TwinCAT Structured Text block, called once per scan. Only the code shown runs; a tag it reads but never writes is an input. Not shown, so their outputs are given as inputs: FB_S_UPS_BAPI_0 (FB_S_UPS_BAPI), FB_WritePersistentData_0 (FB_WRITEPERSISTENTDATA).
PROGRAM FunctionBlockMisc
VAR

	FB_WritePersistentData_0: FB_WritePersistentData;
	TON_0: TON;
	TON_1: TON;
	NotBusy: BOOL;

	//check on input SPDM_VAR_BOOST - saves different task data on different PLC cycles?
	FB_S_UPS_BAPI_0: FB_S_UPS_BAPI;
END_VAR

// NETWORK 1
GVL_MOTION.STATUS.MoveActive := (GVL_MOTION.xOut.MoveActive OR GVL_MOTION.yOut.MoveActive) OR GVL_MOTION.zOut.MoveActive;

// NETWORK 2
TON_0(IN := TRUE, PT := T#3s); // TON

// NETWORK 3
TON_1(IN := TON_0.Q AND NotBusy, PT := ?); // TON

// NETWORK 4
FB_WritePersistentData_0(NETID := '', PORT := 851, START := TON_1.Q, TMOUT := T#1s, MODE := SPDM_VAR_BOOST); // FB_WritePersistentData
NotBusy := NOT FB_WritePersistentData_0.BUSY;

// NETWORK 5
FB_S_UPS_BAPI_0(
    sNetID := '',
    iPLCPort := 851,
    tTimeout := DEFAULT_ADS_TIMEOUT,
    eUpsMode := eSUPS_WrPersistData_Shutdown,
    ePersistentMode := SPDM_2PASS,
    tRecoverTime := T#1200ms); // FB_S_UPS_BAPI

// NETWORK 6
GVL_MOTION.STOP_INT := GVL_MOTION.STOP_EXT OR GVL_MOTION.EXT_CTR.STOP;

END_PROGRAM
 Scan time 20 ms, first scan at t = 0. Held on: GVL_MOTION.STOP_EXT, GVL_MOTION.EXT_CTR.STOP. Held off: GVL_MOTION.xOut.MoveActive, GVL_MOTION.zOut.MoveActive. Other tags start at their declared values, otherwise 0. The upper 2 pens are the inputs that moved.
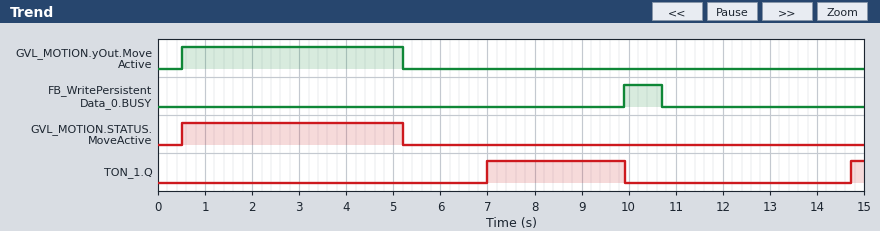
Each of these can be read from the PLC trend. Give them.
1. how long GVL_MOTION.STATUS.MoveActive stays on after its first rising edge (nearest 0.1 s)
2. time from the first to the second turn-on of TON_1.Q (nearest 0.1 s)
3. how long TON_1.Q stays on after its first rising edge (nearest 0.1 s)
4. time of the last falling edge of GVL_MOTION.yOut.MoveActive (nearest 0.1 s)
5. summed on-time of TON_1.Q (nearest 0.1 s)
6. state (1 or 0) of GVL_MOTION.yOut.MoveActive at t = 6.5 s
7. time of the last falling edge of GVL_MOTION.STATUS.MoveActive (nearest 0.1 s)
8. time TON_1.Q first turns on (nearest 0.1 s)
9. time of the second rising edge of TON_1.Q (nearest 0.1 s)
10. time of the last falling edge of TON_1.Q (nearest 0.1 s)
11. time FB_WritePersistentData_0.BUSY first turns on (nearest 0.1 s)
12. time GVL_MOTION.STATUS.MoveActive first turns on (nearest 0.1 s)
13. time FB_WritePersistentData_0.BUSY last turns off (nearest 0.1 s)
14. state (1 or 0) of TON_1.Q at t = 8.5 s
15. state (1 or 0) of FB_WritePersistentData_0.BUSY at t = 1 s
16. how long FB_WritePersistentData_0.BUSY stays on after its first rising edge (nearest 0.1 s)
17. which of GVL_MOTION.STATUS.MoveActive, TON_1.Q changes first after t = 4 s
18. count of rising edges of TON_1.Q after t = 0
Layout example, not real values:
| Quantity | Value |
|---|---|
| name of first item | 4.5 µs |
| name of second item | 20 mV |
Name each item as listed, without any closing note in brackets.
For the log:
| Quantity | Value |
|---|---|
| how long GVL_MOTION.STATUS.MoveActive stays on after its first rising edge | 4.7 s |
| time from the first to the second turn-on of TON_1.Q | 7.7 s |
| how long TON_1.Q stays on after its first rising edge | 2.9 s |
| time of the last falling edge of GVL_MOTION.yOut.MoveActive | 5.2 s |
| summed on-time of TON_1.Q | 3.2 s |
| state (1 or 0) of GVL_MOTION.yOut.MoveActive at t = 6.5 s | 0 |
| time of the last falling edge of GVL_MOTION.STATUS.MoveActive | 5.2 s |
| time TON_1.Q first turns on | 7.0 s |
| time of the second rising edge of TON_1.Q | 14.7 s |
| time of the last falling edge of TON_1.Q | 9.9 s |
| time FB_WritePersistentData_0.BUSY first turns on | 9.9 s |
| time GVL_MOTION.STATUS.MoveActive first turns on | 0.5 s |
| time FB_WritePersistentData_0.BUSY last turns off | 10.7 s |
| state (1 or 0) of TON_1.Q at t = 8.5 s | 1 |
| state (1 or 0) of FB_WritePersistentData_0.BUSY at t = 1 s | 0 |
| how long FB_WritePersistentData_0.BUSY stays on after its first rising edge | 0.8 s |
| which of GVL_MOTION.STATUS.MoveActive, TON_1.Q changes first after t = 4 s | GVL_MOTION.STATUS.MoveActive |
| count of rising edges of TON_1.Q after t = 0 | 2 |
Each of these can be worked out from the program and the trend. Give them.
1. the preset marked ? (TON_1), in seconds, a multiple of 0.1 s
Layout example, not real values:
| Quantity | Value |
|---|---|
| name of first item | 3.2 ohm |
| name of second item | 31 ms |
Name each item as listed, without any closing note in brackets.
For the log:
| Quantity | Value |
|---|---|
| the preset marked ? (TON_1), in seconds, a multiple of 0.1 s | 4.0 s |
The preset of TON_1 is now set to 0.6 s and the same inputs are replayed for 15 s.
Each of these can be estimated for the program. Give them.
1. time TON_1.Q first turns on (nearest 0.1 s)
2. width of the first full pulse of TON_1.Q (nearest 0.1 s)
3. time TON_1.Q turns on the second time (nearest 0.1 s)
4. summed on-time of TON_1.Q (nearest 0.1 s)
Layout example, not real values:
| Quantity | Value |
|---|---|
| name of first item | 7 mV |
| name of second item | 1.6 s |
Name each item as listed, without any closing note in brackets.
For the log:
| Quantity | Value |
|---|---|
| time TON_1.Q first turns on | 3.6 s |
| width of the first full pulse of TON_1.Q | 6.3 s |
| time TON_1.Q turns on the second time | 11.3 s |
| summed on-time of TON_1.Q | 10.0 s |
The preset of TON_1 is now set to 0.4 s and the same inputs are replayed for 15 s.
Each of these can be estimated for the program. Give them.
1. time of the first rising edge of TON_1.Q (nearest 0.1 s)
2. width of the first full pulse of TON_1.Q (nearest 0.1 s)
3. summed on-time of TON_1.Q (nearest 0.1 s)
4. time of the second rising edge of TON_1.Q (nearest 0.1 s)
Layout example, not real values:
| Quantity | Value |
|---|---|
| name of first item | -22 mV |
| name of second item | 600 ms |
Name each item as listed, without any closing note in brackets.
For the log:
| Quantity | Value |
|---|---|
| time of the first rising edge of TON_1.Q | 3.4 s |
| width of the first full pulse of TON_1.Q | 6.5 s |
| summed on-time of TON_1.Q | 10.4 s |
| time of the second rising edge of TON_1.Q | 11.1 s |
